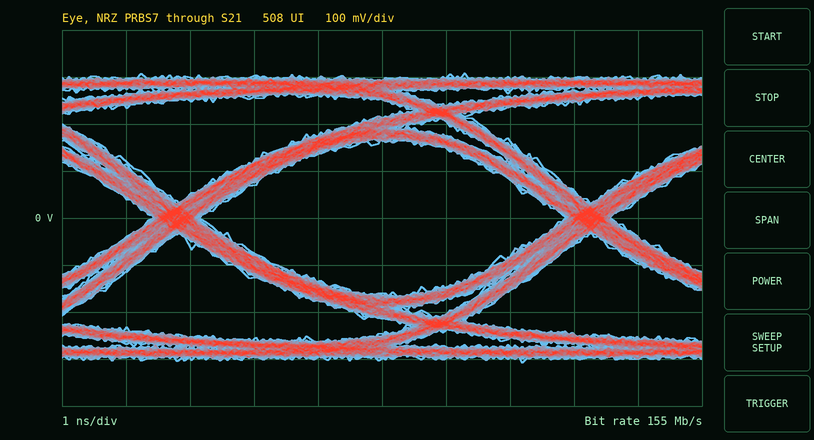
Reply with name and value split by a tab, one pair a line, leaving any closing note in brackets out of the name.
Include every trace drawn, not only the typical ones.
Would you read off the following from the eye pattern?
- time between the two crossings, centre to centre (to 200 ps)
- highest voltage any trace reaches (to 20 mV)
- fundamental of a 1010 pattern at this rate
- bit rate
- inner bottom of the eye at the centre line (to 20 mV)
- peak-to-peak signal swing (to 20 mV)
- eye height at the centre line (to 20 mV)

time between the two crossings, centre to centre	6.4 ns
highest voltage any trace reaches	300 mV
fundamental of a 1010 pattern at this rate	77.5 MHz
bit rate	155 Mb/s
inner bottom of the eye at the centre line	-160 mV
peak-to-peak signal swing	620 mV
eye height at the centre line	320 mV
